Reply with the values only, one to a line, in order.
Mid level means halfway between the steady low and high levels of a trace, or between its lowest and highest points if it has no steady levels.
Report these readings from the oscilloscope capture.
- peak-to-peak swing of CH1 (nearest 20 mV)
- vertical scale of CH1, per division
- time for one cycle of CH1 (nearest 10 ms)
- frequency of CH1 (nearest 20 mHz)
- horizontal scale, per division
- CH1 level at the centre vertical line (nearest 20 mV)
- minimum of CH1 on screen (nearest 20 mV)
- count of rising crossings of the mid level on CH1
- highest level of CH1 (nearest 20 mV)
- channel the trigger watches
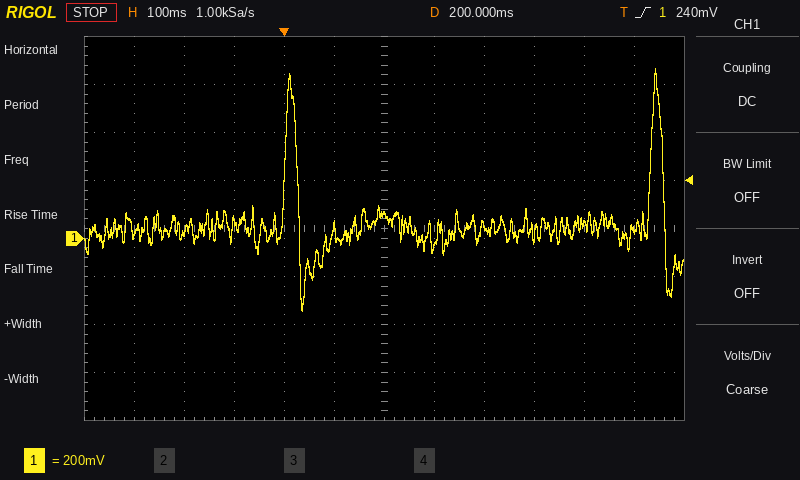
1.00 V
200 mV
730 ms
1.36 Hz
100 ms
100 mV
-300 mV
2
700 mV
CH1
